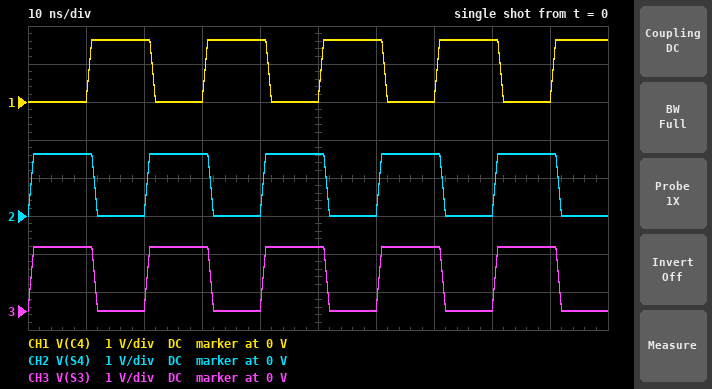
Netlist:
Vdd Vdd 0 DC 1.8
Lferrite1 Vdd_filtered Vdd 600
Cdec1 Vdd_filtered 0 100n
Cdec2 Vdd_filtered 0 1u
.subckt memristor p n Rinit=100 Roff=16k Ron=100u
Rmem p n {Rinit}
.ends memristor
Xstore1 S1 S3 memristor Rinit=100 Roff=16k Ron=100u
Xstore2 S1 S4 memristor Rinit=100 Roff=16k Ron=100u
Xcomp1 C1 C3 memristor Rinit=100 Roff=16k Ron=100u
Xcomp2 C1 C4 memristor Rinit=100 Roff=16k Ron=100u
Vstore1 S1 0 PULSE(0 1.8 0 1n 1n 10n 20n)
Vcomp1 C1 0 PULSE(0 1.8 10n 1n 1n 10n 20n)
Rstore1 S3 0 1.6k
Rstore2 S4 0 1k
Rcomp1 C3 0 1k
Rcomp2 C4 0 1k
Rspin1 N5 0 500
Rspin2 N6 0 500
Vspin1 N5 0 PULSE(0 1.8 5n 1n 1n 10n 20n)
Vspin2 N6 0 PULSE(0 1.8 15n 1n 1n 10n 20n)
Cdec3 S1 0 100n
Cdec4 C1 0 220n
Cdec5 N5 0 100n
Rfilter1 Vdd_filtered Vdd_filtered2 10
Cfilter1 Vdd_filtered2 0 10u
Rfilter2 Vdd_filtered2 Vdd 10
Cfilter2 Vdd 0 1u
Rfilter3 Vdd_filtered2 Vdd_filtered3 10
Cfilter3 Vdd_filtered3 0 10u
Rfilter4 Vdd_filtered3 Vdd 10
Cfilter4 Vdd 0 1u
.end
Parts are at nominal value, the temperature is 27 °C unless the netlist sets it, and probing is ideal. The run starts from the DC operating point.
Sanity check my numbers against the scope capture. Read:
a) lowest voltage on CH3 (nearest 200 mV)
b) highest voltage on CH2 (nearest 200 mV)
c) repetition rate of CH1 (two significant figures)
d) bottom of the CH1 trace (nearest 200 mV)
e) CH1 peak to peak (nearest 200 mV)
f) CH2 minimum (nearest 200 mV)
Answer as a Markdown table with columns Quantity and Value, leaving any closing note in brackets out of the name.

| Quantity | Value |
|---|---|
| lowest voltage on CH3 | 0 V |
| highest voltage on CH2 | 1.6 V |
| repetition rate of CH1 | 50 MHz |
| bottom of the CH1 trace | 0 V |
| CH1 peak to peak | 1.6 V |
| CH2 minimum | 0 V |
